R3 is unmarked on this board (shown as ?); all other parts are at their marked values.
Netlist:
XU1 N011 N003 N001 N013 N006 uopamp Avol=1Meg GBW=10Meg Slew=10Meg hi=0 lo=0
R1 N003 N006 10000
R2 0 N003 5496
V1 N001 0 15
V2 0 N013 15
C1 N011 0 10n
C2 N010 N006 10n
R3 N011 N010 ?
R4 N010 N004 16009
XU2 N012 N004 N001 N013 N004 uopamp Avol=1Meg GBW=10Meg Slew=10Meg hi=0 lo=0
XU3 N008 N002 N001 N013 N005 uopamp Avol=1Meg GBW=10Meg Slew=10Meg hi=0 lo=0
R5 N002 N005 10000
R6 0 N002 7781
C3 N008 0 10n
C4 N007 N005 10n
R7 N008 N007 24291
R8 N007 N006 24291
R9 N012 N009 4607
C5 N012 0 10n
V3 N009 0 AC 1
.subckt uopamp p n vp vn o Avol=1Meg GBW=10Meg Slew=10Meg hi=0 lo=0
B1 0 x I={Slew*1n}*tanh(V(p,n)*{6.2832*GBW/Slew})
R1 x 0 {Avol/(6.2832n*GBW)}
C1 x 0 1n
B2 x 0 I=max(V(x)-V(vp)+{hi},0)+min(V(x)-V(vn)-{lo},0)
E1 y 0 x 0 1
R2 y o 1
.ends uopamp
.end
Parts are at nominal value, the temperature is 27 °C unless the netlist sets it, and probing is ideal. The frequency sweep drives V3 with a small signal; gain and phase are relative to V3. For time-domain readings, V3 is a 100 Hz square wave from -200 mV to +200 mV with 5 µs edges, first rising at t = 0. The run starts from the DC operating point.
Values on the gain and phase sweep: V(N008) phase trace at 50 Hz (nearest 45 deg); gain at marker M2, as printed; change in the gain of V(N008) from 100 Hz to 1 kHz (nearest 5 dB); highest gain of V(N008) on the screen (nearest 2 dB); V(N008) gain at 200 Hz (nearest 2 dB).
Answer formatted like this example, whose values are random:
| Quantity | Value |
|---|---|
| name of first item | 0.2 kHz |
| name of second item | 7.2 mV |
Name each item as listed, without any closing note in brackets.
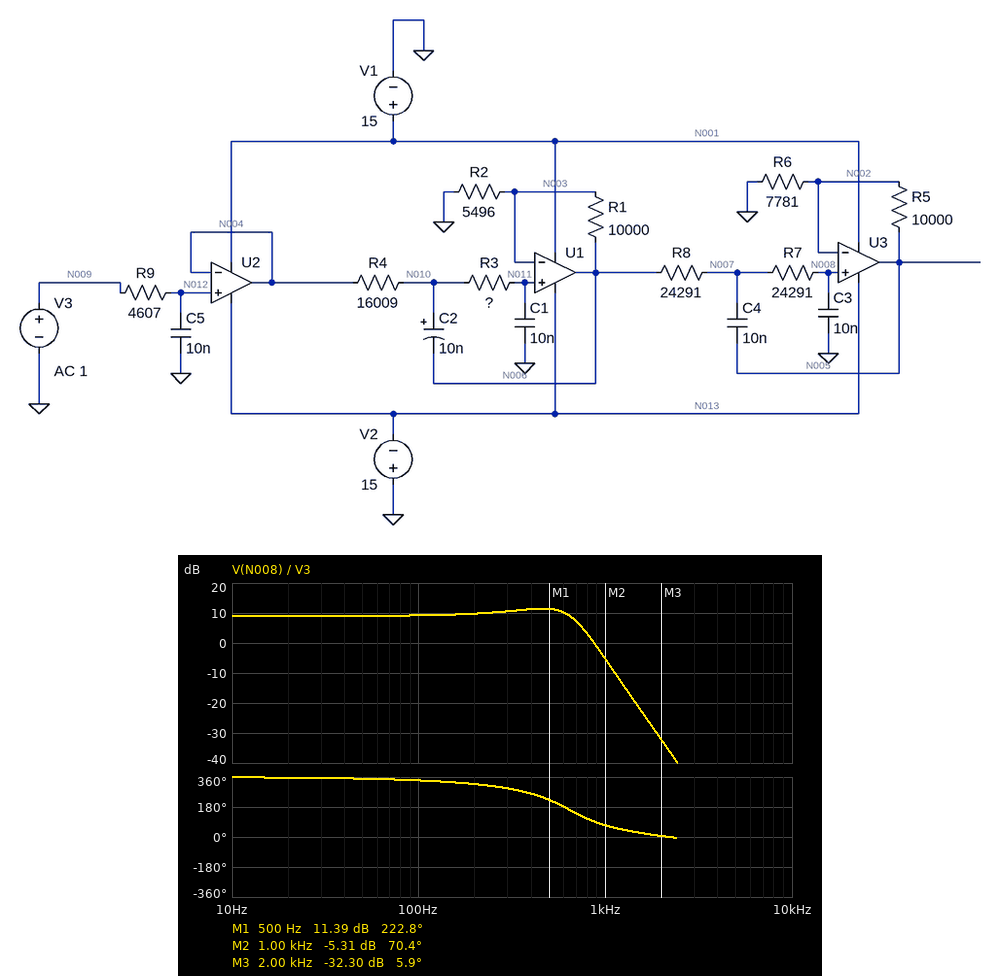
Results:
| Quantity | Value |
|---|---|
| V(N008) phase trace at 50 Hz | 360 deg |
| gain at marker M2, as printed | -5.31 dB |
| change in the gain of V(N008) from 100 Hz to 1 kHz | -15 dB |
| highest gain of V(N008) on the screen | 12 dB |
| V(N008) gain at 200 Hz | 10 dB |
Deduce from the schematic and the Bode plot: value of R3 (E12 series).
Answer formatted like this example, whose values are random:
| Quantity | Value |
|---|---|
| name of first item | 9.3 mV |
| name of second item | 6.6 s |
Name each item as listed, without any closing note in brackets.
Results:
| Quantity | Value |
|---|---|
| value of R3 | 47 kΩ |
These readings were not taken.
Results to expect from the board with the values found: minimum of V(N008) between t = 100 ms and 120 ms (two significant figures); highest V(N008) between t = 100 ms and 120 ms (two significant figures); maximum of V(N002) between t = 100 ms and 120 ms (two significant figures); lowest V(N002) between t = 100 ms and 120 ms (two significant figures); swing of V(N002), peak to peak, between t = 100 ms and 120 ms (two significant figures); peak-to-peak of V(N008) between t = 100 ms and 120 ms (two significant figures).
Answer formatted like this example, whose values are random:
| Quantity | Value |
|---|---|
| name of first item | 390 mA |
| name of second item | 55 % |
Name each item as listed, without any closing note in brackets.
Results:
| Quantity | Value |
|---|---|
| minimum of V(N008) between t = 100 ms and 120 ms | -880 mV |
| highest V(N008) between t = 100 ms and 120 ms | 880 mV |
| maximum of V(N002) between t = 100 ms and 120 ms | 880 mV |
| lowest V(N002) between t = 100 ms and 120 ms | -880 mV |
| swing of V(N002), peak to peak, between t = 100 ms and 120 ms | 1.8 V |
| peak-to-peak of V(N008) between t = 100 ms and 120 ms | 1.8 V |
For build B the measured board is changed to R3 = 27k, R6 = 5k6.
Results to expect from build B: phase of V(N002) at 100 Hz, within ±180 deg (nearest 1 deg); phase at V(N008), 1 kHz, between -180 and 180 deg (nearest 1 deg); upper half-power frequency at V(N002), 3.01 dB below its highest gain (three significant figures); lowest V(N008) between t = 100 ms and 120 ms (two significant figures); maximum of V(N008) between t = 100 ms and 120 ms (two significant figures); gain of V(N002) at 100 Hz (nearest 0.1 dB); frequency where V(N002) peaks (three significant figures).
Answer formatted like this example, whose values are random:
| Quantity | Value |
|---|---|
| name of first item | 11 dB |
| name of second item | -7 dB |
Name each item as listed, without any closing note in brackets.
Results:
| Quantity | Value |
|---|---|
| phase of V(N002) at 100 Hz, within ±180 deg | -9 deg |
| phase at V(N008), 1 kHz, between -180 and 180 deg | 49 deg |
| upper half-power frequency at V(N002), 3.01 dB below its highest gain | 713 Hz |
| lowest V(N008) between t = 100 ms and 120 ms | -1.7 V |
| maximum of V(N008) between t = 100 ms and 120 ms | 1.7 V |
| gain of V(N002) at 100 Hz | 9.3 dB |
| frequency where V(N002) peaks | 649 Hz |
